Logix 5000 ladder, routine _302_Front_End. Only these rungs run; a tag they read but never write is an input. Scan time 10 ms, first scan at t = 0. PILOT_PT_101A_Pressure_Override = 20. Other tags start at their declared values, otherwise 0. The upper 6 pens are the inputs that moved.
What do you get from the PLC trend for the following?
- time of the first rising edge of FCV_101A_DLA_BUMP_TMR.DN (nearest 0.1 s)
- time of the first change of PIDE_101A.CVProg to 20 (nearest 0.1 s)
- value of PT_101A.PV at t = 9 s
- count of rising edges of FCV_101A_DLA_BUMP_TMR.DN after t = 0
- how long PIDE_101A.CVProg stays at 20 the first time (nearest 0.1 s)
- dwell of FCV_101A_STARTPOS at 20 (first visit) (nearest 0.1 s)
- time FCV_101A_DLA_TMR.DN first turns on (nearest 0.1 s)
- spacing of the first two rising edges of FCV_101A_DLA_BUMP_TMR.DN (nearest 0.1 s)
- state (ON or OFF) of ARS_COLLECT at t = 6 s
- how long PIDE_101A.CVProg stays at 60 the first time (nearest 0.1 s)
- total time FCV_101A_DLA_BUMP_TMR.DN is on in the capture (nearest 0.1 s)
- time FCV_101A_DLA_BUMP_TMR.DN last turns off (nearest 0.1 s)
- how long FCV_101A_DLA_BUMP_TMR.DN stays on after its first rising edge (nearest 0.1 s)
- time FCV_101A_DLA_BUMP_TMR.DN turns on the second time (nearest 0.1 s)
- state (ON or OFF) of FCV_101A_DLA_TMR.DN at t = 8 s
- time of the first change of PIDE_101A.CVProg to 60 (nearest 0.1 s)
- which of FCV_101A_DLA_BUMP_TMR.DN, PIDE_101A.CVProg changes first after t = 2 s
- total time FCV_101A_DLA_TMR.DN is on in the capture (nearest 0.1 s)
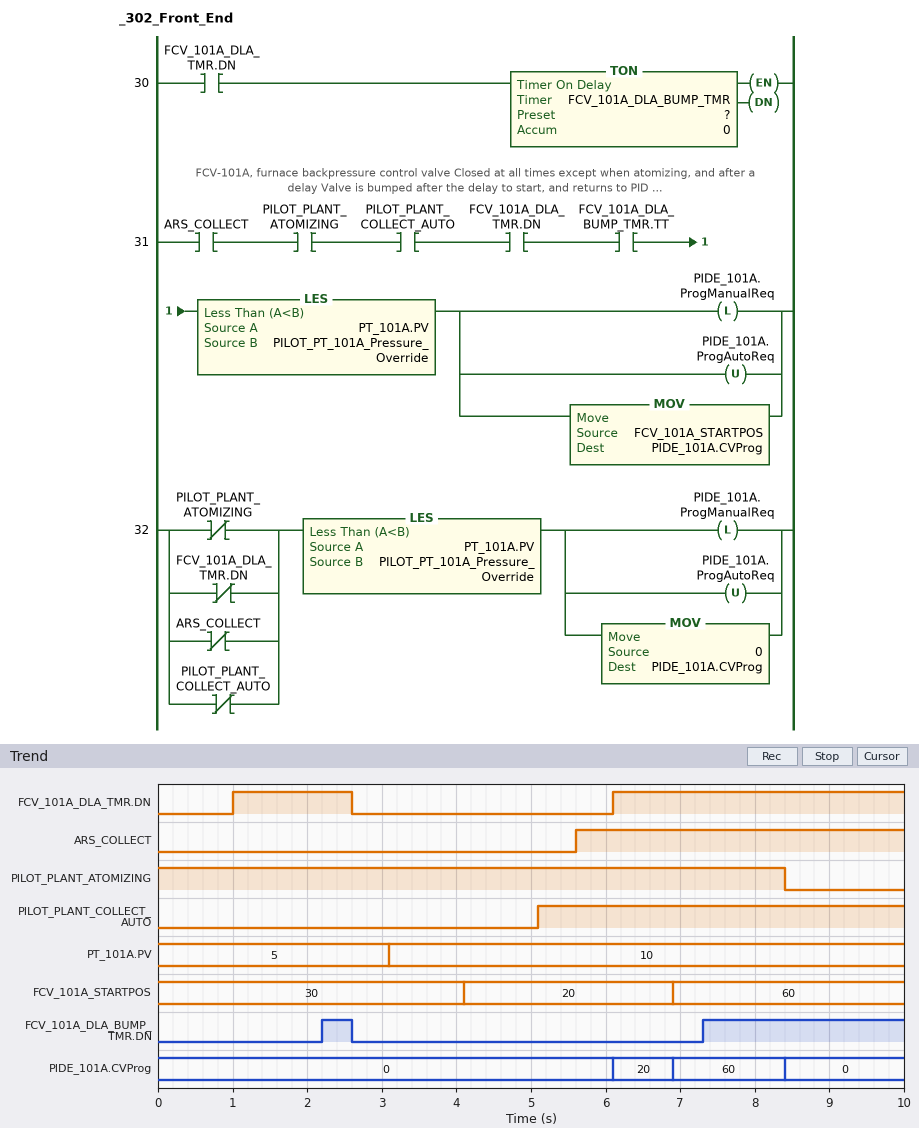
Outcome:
2.2 s
6.1 s
10
2
0.8 s
2.8 s
1.0 s
5.1 s
ON
1.5 s
3.1 s
2.6 s
0.4 s
7.3 s
ON
6.9 s
FCV_101A_DLA_BUMP_TMR.DN
5.5 s
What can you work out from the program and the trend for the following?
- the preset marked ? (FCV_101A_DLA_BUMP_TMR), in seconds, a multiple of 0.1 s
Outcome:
1.2 s
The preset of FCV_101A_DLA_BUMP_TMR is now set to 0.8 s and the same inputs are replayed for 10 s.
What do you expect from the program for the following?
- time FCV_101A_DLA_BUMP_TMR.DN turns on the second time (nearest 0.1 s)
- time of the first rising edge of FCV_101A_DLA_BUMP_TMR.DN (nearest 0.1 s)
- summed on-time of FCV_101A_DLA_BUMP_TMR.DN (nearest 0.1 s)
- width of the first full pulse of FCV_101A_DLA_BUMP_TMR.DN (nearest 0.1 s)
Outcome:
6.9 s
1.8 s
3.9 s
0.8 s
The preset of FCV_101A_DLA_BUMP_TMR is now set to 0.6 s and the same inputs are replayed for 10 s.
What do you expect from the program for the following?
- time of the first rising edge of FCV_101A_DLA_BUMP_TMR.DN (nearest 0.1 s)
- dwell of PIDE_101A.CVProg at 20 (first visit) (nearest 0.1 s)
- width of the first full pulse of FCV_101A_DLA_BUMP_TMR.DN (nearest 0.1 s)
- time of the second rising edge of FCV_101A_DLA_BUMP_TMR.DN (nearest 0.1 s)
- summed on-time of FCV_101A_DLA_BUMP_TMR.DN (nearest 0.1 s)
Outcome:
1.6 s
2.3 s
1.0 s
6.7 s
4.3 s
